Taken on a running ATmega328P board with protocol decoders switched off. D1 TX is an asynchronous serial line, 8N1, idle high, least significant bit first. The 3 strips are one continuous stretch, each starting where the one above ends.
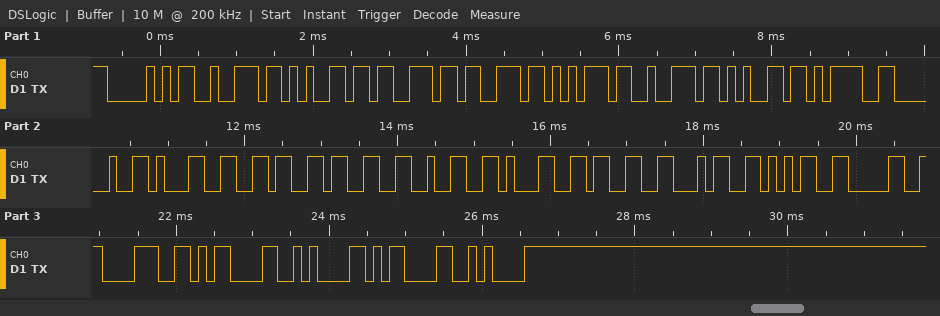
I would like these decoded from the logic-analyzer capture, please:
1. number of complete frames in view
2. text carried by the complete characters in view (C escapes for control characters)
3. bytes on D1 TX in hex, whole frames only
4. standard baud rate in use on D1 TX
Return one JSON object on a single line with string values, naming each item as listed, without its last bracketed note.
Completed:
{"number of complete frames in view": "24", "text carried by the complete characters in view": "\"Pressure= 1632134508\\r\\n\\r\\n\"", "bytes on D1 TX in hex, whole frames only": "50 72 65 73 73 75 72 65 3D 20 31 36 33 32 31 33 34 35 30 38 0D 0A 0D 0A", "standard baud rate in use on D1 TX": "9600 baud"}
